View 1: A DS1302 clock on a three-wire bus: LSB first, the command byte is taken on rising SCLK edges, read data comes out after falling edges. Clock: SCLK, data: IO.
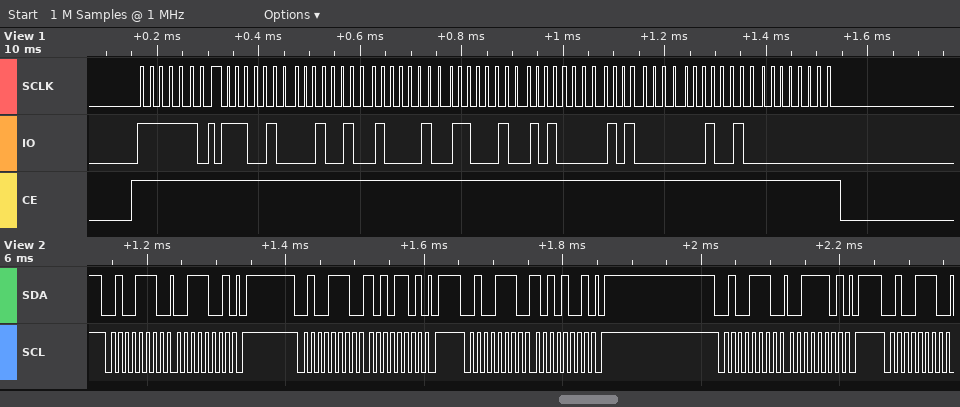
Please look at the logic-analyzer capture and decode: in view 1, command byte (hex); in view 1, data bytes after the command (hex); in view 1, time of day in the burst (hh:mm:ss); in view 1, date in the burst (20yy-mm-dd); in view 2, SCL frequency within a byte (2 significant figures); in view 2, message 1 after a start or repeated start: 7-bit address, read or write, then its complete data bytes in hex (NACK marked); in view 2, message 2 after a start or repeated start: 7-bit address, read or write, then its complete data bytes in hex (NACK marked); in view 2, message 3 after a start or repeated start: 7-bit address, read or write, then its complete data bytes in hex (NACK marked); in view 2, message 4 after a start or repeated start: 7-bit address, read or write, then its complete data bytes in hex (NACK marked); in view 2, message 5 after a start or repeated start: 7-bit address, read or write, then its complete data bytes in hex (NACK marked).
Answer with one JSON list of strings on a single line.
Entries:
["0xBF", "27 24 21 23 05 05 24 00", "21:24:27", "2024-05-23", "100 kHz", "0x27 write: 39", "0x27 write: AD", "0x27 write: A9", "0x27 write: 3D", "0x27 write"]
